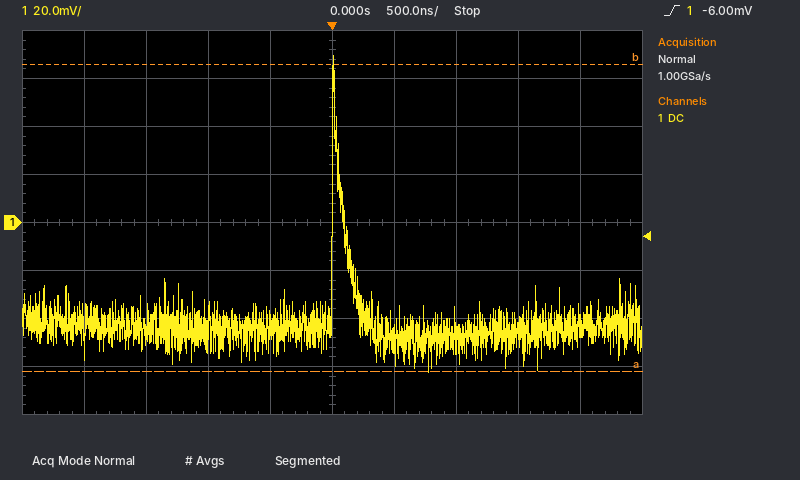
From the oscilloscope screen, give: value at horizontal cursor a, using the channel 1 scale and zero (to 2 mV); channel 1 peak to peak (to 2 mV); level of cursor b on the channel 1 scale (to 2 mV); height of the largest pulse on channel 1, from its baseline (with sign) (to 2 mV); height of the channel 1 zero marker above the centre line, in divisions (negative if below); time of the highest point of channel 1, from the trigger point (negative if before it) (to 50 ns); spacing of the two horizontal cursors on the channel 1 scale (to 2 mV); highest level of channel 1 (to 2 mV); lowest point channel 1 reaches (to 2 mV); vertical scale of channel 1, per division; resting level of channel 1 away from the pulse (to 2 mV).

-62 mV
132 mV
66 mV
+114 mV
0.0 div
0 ns
128 mV
70 mV
-62 mV
20 mV
-44 mV
